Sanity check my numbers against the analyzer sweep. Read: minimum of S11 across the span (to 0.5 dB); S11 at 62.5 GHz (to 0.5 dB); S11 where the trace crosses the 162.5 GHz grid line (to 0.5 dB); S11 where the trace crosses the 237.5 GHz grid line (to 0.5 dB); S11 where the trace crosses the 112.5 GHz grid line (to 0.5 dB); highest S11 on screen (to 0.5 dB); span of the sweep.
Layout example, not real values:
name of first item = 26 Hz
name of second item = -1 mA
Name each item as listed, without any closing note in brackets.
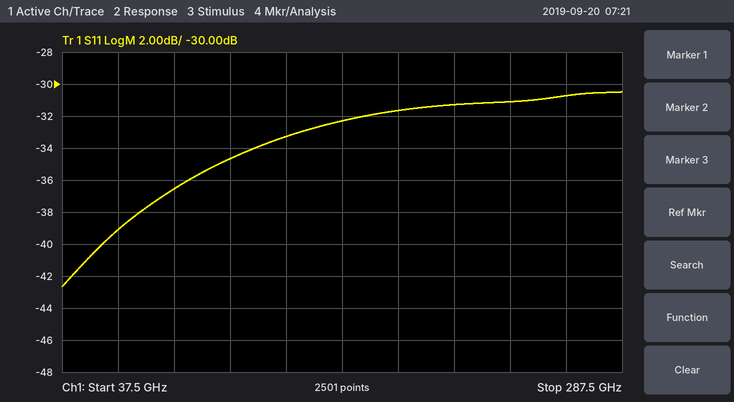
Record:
minimum of S11 across the span = -42.5 dB
S11 at 62.5 GHz = -39.0 dB
S11 where the trace crosses the 162.5 GHz grid line = -32.5 dB
S11 where the trace crosses the 237.5 GHz grid line = -31.0 dB
S11 where the trace crosses the 112.5 GHz grid line = -34.5 dB
highest S11 on screen = -30.5 dB
span of the sweep = 250 GHz
